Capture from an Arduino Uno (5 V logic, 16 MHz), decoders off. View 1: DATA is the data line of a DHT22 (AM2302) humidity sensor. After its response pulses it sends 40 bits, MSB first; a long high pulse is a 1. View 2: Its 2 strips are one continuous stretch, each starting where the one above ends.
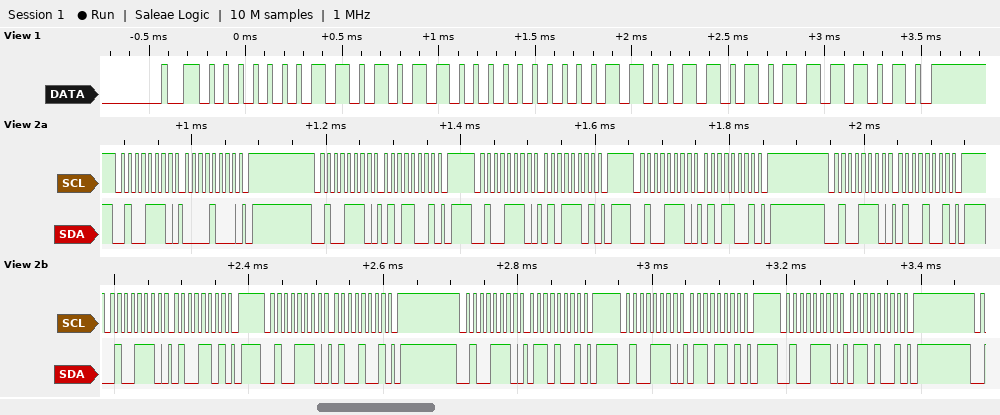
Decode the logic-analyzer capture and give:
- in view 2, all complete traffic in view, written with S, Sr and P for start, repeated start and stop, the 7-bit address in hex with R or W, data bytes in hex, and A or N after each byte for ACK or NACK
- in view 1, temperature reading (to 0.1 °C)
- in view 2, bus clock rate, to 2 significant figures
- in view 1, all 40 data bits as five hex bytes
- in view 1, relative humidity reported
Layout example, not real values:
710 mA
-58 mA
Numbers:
S 27W A 08 A P S 27W A 59 A P S 27W A 5D A P S 27W A 59 A P S 27W A 49 A P S 27W A 4D A P S 27W A 49 A P S 27W A 69 A P S 27W A 6D A P S 27W A 69 A P
20.5 °C
100 kHz
01 AC 00 CD 7A
42.8 %
